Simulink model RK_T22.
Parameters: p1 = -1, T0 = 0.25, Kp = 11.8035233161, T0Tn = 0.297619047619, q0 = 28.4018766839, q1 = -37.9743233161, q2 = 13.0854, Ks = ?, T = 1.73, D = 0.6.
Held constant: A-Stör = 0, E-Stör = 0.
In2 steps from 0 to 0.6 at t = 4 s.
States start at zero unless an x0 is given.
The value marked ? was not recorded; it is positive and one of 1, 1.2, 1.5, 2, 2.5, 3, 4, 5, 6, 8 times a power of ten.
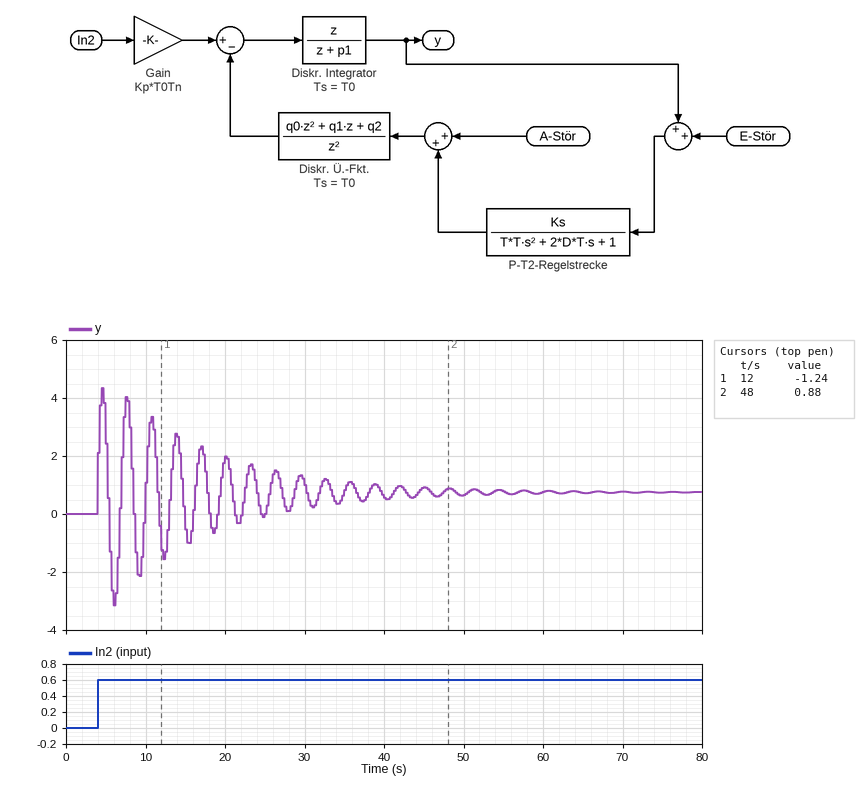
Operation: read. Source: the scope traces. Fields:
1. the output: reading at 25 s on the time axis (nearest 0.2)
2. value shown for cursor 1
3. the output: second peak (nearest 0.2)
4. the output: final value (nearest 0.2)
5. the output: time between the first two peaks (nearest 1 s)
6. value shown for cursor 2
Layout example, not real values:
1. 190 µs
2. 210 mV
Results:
1. 0.0
2. -1.24
3. 4.0
4. 0.8
5. 3 s
6. 0.88
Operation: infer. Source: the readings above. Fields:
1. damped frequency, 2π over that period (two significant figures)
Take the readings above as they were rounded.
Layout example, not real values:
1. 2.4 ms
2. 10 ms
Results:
1. 2.1 rad/s
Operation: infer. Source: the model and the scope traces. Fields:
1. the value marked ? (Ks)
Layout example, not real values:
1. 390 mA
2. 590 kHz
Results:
1. 0.8
